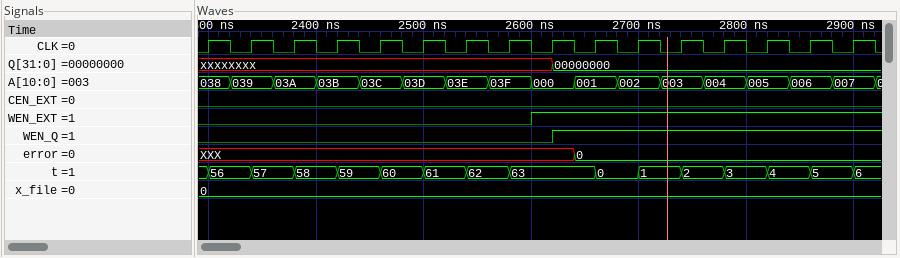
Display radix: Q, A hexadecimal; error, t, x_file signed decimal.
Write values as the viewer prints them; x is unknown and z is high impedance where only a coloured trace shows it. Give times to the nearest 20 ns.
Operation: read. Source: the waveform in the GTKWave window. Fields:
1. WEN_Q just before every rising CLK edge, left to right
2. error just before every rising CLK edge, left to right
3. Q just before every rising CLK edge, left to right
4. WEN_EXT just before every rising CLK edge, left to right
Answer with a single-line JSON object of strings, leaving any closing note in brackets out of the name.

{"WEN_Q just before every rising CLK edge, left to right": "0 0 0 0 0 0 0 0 0 1 1 1 1 1 1 1", "error just before every rising CLK edge, left to right": "XXX, XXX, XXX, XXX, XXX, XXX, XXX, XXX, XXX, 0, 0, 0, 0, 0, 0, 0", "Q just before every rising CLK edge, left to right": "xxxxxxxx, xxxxxxxx, xxxxxxxx, xxxxxxxx, xxxxxxxx, xxxxxxxx, xxxxxxxx, xxxxxxxx, xxxxxxxx, 00000000, 00000000, 00000000, 00000000, 00000000, 00000000, 00000000", "WEN_EXT just before every rising CLK edge, left to right": "0 0 0 0 0 0 0 0 1 1 1 1 1 1 1 1"}
